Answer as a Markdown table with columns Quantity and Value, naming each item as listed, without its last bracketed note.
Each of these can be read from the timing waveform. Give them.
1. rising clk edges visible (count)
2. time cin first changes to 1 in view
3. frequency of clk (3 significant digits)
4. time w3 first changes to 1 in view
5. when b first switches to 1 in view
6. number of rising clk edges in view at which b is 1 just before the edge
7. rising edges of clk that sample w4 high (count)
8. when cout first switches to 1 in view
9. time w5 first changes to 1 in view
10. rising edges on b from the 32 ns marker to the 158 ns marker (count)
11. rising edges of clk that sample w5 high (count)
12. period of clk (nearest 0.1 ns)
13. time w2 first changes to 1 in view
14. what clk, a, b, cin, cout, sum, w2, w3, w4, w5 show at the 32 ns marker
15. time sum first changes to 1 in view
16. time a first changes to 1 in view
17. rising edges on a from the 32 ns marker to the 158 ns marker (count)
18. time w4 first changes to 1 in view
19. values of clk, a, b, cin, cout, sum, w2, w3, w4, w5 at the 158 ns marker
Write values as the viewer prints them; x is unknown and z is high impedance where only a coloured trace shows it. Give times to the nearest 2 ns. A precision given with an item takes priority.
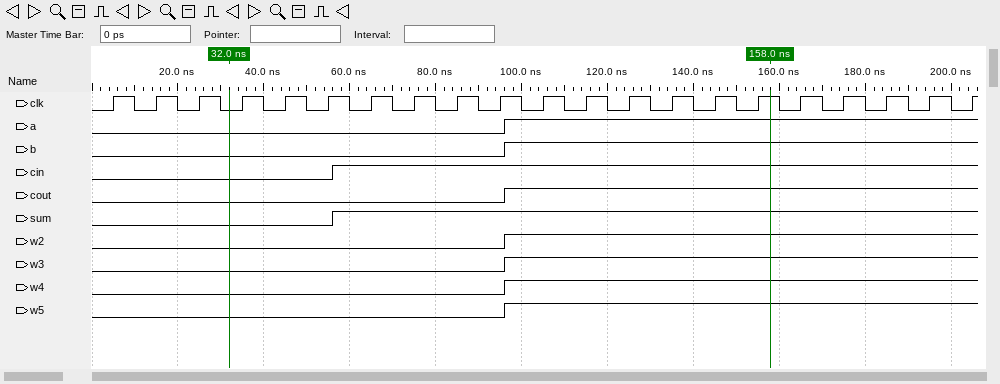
| Quantity | Value |
|---|---|
| rising clk edges visible | 21 |
| time cin first changes to 1 in view | 56 ns |
| frequency of clk | 100 MHz |
| time w3 first changes to 1 in view | 96 ns |
| when b first switches to 1 in view | 96 ns |
| number of rising clk edges in view at which b is 1 just before the edge | 11 |
| rising edges of clk that sample w4 high | 11 |
| when cout first switches to 1 in view | 96 ns |
| time w5 first changes to 1 in view | 96 ns |
| rising edges on b from the 32 ns marker to the 158 ns marker | 1 |
| rising edges of clk that sample w5 high | 11 |
| period of clk | 10 ns |
| time w2 first changes to 1 in view | 96 ns |
| what clk, a, b, cin, cout, sum, w2, w3, w4, w5 show at the 32 ns marker | clk=0, a=0, b=0, cin=0, cout=0, sum=0, w2=0, w3=0, w4=0, w5=0 |
| time sum first changes to 1 in view | 56 ns |
| time a first changes to 1 in view | 96 ns |
| rising edges on a from the 32 ns marker to the 158 ns marker | 1 |
| time w4 first changes to 1 in view | 96 ns |
| values of clk, a, b, cin, cout, sum, w2, w3, w4, w5 at the 158 ns marker | clk=1, a=1, b=1, cin=1, cout=1, sum=1, w2=1, w3=1, w4=1, w5=1 |
